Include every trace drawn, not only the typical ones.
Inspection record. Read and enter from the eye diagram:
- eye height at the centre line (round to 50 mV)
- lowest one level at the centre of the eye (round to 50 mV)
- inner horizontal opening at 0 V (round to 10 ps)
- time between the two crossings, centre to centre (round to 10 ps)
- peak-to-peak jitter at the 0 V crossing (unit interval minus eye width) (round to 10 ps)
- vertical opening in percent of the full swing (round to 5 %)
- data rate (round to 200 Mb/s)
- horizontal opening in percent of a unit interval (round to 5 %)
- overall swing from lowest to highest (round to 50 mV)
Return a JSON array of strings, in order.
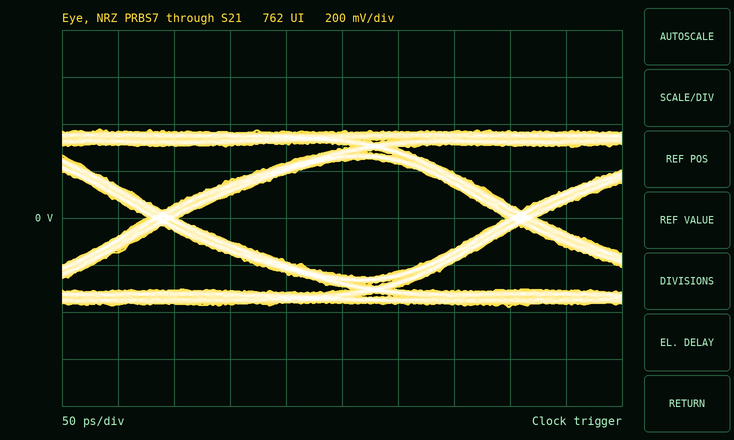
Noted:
["500 mV", "250 mV", "290 ps", "320 ps", "30 ps", "65 %", "3.2 Gb/s", "90 %", "750 mV"]
